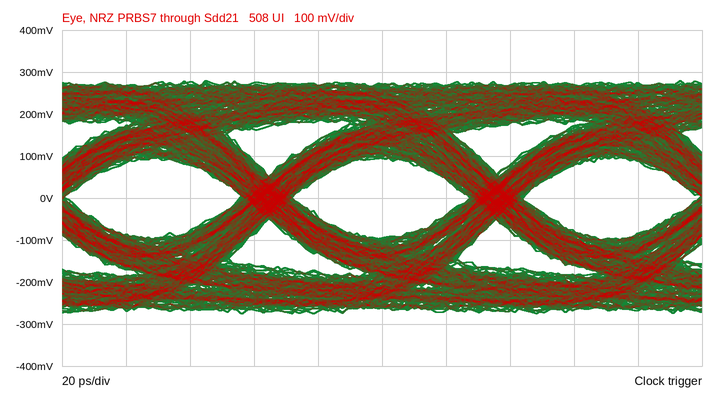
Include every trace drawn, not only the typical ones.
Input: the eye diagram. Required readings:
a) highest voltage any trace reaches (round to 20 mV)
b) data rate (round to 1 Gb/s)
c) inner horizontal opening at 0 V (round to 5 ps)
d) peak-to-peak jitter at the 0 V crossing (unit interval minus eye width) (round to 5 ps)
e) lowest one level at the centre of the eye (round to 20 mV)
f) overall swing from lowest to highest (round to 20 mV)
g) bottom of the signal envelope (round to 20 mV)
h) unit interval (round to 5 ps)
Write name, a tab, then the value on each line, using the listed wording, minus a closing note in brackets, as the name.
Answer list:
highest voltage any trace reaches	280 mV
data rate	14 Gb/s
inner horizontal opening at 0 V	55 ps
peak-to-peak jitter at the 0 V crossing (unit interval minus eye width)	15 ps
lowest one level at the centre of the eye	100 mV
overall swing from lowest to highest	560 mV
bottom of the signal envelope	-280 mV
unit interval	70 ps
